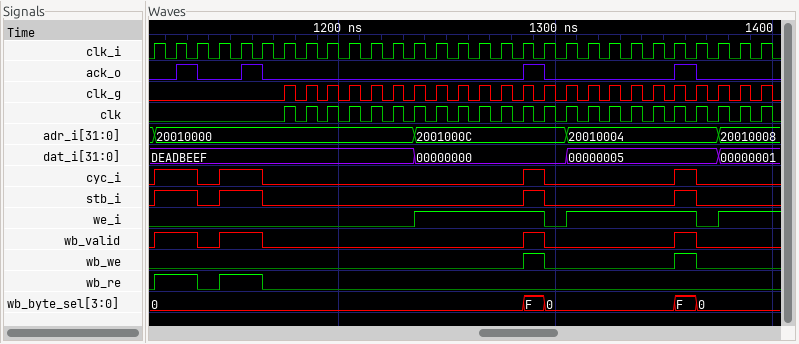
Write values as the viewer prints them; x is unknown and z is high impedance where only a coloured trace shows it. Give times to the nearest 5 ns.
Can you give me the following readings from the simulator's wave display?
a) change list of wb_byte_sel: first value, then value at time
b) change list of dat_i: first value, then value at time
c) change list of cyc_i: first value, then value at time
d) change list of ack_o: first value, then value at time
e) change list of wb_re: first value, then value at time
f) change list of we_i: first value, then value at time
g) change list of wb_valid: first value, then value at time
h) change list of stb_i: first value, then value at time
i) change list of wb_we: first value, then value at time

0, F at 1285 ns, 0 at 1295 ns, F at 1355 ns, 0 at 1365 ns
DEADBEEF, 00000000 at 1235 ns, 00000005 at 1305 ns, 00000001 at 1375 ns
0, 1 at 1115 ns, 0 at 1135 ns, 1 at 1145 ns, 0 at 1165 ns, 1 at 1285 ns, 0 at 1295 ns, 1 at 1355 ns, 0 at 1365 ns
0, 1 at 1125 ns, 0 at 1135 ns, 1 at 1155 ns, 0 at 1165 ns, 1 at 1285 ns, 0 at 1295 ns, 1 at 1355 ns, 0 at 1365 ns
0, 1 at 1115 ns, 0 at 1135 ns, 1 at 1145 ns, 0 at 1165 ns
0, 1 at 1235 ns, 0 at 1295 ns, 1 at 1305 ns, 0 at 1365 ns, 1 at 1375 ns
0, 1 at 1115 ns, 0 at 1135 ns, 1 at 1145 ns, 0 at 1165 ns, 1 at 1285 ns, 0 at 1295 ns, 1 at 1355 ns, 0 at 1365 ns
0, 1 at 1115 ns, 0 at 1135 ns, 1 at 1145 ns, 0 at 1165 ns, 1 at 1285 ns, 0 at 1295 ns, 1 at 1355 ns, 0 at 1365 ns
0, 1 at 1285 ns, 0 at 1295 ns, 1 at 1355 ns, 0 at 1365 ns
